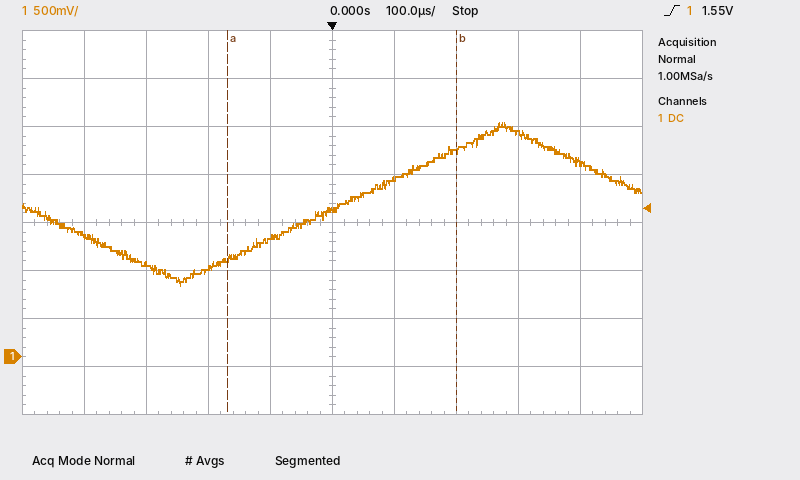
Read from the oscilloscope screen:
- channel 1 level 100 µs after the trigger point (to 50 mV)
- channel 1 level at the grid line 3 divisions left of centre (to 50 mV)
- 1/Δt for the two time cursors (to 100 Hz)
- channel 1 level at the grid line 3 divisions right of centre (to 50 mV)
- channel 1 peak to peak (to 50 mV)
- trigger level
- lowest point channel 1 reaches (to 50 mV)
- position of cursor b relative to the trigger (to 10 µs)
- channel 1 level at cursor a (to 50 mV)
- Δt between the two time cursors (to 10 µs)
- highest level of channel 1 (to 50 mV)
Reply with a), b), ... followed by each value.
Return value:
a) 1.85 V
b) 950 mV
c) 2.7 kHz
d) 2.35 V
e) 1.70 V
f) 1.55 V
g) 750 mV
h) +200 µs
i) 1.05 V
j) 370 µs
k) 2.45 V
